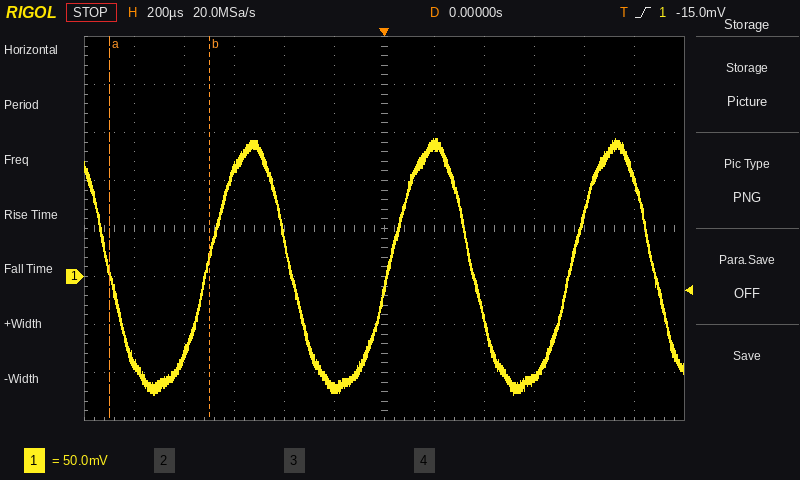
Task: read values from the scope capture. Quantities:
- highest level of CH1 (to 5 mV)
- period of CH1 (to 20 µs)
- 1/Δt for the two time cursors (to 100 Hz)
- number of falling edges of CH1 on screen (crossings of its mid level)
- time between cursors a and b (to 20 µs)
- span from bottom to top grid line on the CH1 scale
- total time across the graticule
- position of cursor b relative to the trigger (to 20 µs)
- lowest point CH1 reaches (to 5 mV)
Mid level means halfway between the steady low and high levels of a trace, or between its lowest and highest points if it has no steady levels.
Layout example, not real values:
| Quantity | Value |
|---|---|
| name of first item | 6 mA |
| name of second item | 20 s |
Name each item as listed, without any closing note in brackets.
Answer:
| Quantity | Value |
|---|---|
| highest level of CH1 | 145 mV |
| period of CH1 | 720 µs |
| 1/Δt for the two time cursors | 2.5 kHz |
| number of falling edges of CH1 on screen | 4 |
| time between cursors a and b | 400 µs |
| span from bottom to top grid line on the CH1 scale | 400 mV |
| total time across the graticule | 2.4 ms |
| position of cursor b relative to the trigger | -700 µs |
| lowest point CH1 reaches | -125 mV |
